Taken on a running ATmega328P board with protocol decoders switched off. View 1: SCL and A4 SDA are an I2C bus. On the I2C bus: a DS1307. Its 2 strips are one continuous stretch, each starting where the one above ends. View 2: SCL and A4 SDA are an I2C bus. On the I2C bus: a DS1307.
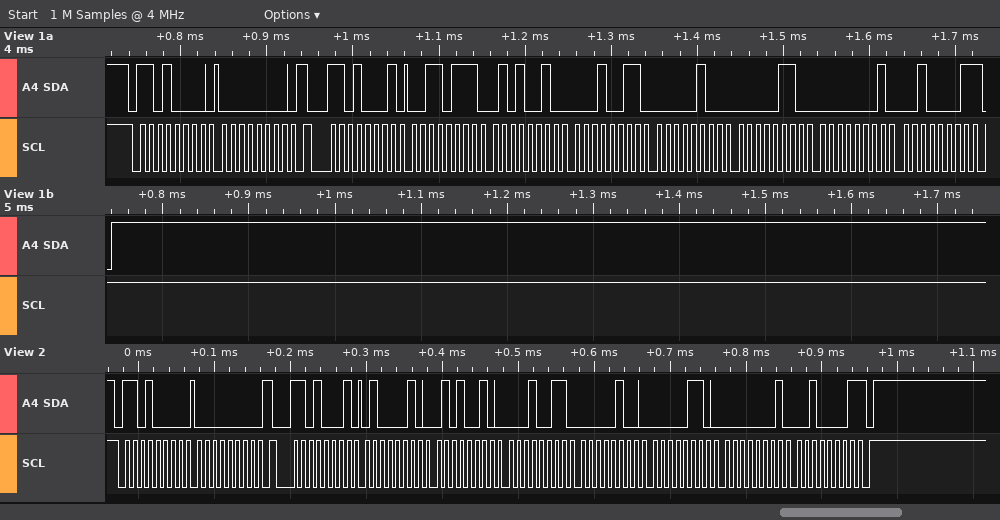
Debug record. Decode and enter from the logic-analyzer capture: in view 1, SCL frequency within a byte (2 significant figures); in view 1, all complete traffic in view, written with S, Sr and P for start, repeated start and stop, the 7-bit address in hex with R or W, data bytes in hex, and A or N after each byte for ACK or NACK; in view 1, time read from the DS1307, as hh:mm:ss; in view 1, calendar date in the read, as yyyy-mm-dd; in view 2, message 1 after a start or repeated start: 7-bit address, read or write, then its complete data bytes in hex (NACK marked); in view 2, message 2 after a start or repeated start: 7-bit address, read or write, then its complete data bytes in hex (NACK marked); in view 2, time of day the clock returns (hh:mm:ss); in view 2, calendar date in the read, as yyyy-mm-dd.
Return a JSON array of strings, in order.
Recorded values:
["100 kHz", "S 68W A 00 A Sr 68R A 37 A 52 A 13 A 04 A 06 A 01 A 21 N P", "13:52:37", "2021-01-06", "0x68 write: 00", "0x68 read: 42 52 13 04 06 01 21 NACK", "13:52:42", "2021-01-06"]
